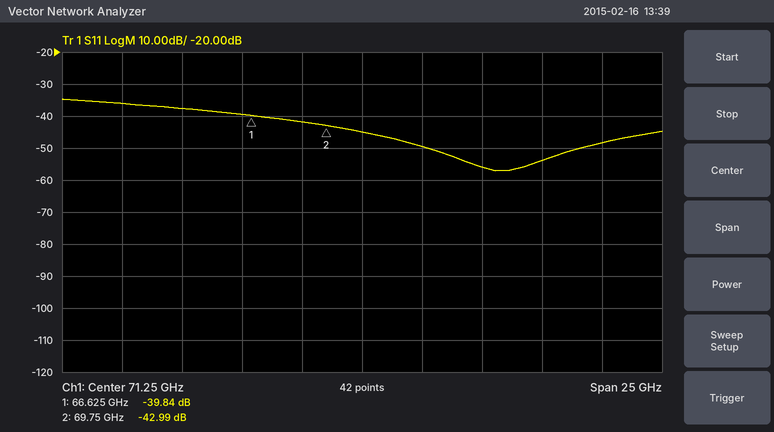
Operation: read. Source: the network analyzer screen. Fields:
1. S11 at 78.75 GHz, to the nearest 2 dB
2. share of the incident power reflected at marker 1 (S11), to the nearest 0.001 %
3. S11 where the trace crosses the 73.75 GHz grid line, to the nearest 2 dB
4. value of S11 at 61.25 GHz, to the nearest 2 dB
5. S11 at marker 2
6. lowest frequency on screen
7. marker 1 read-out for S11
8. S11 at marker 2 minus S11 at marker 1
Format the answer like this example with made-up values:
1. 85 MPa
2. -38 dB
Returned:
1. -54 dB
2. 0.010 %
3. -50 dB
4. -36 dB
5. -42.99 dB
6. 58.75 GHz
7. -39.84 dB
8. -3.15 dB
